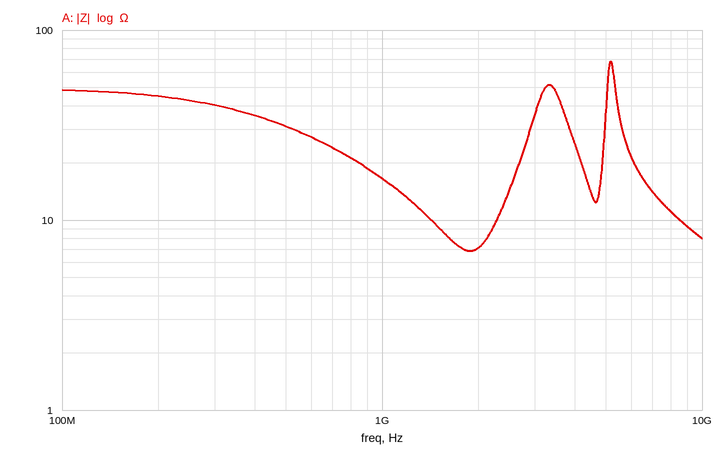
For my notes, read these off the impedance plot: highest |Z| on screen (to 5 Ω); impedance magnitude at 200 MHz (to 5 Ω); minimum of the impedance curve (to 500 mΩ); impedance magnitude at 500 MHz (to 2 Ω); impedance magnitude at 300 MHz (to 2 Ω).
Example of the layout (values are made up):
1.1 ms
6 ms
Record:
70 Ω
45 Ω
7.0 Ω
32 Ω
40 Ω
